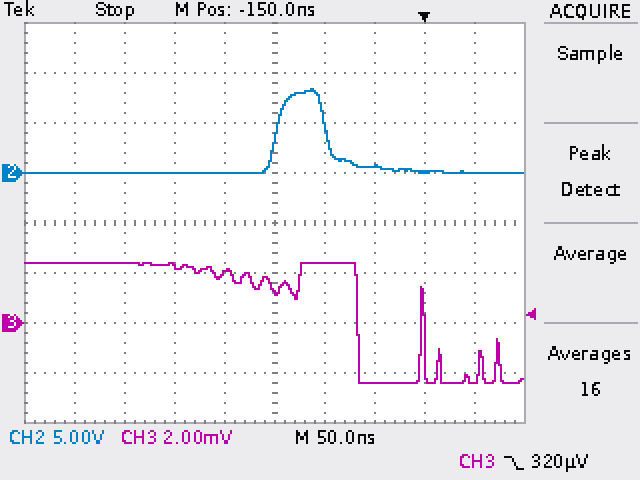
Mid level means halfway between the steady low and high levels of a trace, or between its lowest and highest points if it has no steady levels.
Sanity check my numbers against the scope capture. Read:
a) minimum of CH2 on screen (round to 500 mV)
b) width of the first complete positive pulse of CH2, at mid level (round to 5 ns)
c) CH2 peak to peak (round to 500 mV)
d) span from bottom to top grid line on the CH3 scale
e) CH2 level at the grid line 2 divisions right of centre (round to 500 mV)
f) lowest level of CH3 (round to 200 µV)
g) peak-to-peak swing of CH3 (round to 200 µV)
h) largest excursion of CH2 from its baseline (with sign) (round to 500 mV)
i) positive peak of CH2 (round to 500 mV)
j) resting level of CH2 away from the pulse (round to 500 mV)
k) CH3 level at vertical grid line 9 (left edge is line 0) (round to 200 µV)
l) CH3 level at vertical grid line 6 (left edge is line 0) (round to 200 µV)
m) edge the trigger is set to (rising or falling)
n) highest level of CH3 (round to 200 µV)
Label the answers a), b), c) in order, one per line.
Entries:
a) 0.0 V
b) 50 ns
c) 8.5 V
d) 16 mV
e) 500 mV
f) -2.4 mV
g) 4.8 mV
h) +8.5 V
i) 8.5 V
j) 0.0 V
k) -2.2 mV
l) 2.4 mV
m) falling
n) 2.4 mV
